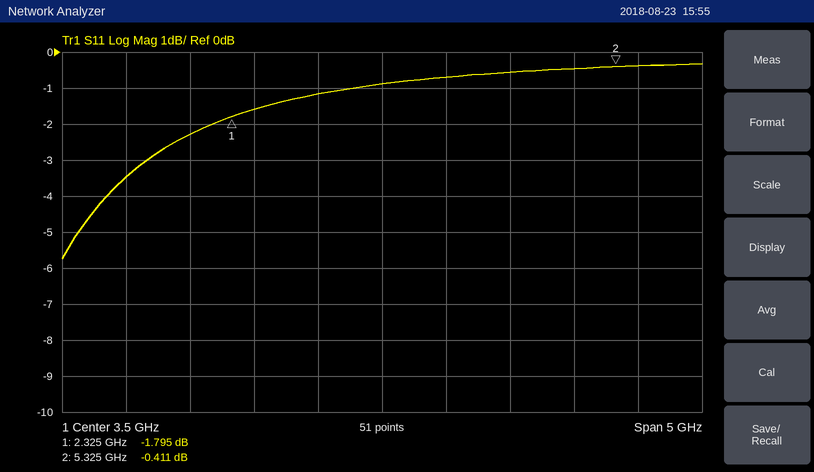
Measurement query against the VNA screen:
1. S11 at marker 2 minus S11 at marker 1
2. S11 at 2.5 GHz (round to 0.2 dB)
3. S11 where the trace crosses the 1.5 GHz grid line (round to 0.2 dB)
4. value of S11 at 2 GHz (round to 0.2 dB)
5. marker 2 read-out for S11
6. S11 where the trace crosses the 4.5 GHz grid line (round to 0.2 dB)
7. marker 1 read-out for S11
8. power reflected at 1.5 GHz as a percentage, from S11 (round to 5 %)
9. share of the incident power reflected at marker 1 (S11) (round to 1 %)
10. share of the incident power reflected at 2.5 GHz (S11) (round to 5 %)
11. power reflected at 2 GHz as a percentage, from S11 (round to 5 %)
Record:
1.384 dB
-1.6 dB
-3.4 dB
-2.2 dB
-0.411 dB
-0.6 dB
-1.795 dB
45 %
66 %
70 %
60 %
